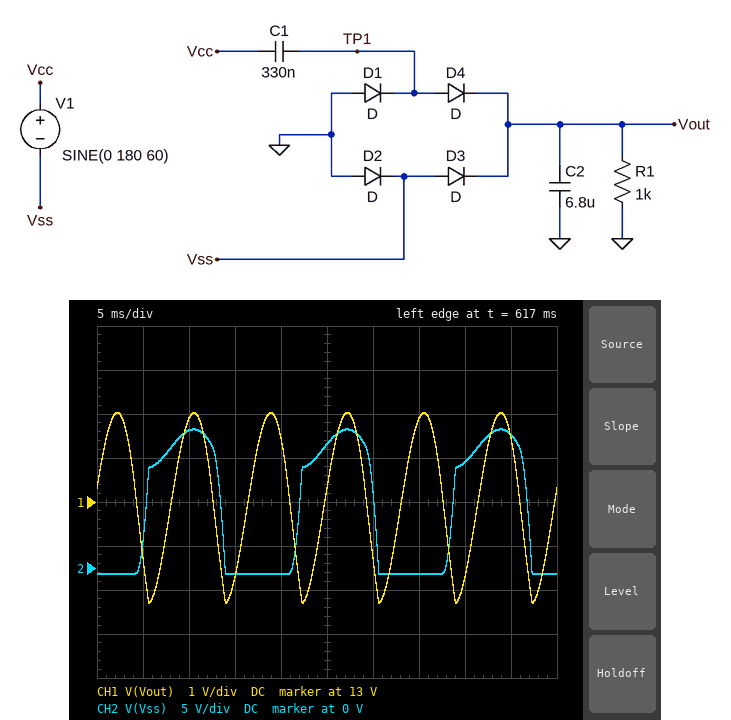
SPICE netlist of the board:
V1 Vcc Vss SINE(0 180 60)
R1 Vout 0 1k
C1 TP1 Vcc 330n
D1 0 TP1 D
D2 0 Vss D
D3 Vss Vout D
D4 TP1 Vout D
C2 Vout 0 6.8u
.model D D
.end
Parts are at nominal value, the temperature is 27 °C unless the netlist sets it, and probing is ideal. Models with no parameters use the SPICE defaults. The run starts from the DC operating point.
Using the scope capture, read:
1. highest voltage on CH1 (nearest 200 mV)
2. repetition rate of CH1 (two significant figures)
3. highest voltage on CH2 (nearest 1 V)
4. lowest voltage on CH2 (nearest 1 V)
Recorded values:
15.0 V
120 Hz
16 V
-1 V
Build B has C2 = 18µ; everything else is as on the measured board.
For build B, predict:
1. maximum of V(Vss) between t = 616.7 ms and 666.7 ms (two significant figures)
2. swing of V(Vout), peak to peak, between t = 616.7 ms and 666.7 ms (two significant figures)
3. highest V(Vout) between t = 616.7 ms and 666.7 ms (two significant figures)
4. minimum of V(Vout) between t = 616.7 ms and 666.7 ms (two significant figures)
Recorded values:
15 V
1.7 V
14 V
12 V
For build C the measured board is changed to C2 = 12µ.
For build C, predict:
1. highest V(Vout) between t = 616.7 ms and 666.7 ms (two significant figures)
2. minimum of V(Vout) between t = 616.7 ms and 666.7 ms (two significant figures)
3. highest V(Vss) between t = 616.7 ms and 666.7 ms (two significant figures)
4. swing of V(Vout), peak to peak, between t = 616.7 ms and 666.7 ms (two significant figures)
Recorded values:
14 V
12 V
15 V
2.5 V
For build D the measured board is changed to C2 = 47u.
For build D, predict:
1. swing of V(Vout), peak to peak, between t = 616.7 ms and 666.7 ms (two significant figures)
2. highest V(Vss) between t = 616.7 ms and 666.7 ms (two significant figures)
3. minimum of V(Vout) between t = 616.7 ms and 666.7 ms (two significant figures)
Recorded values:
650 mV
14 V
13 V
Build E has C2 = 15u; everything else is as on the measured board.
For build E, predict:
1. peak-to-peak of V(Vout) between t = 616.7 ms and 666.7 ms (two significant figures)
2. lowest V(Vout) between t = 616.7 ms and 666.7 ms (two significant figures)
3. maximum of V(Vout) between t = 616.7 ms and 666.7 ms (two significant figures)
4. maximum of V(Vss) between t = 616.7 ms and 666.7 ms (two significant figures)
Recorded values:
2.0 V
12 V
14 V
15 V
